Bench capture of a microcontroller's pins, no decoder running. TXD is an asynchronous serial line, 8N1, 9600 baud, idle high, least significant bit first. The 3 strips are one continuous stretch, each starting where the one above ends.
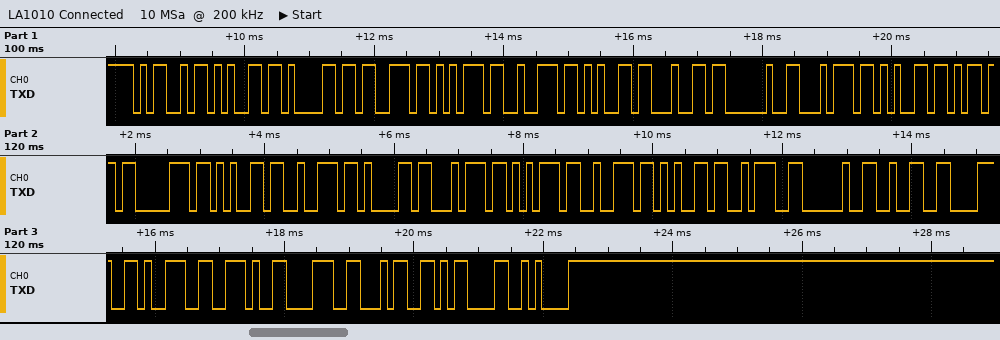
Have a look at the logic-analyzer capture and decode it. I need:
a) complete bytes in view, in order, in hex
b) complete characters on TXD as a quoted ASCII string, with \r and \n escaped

4D 65 61 73 75 72 65 64 20 74 65 6D 70 65 72 61 74 75 72 65 3A 20 32 38 39 2E 38 34 0D 0A
"Measured temperature: 289.84\r\n"
